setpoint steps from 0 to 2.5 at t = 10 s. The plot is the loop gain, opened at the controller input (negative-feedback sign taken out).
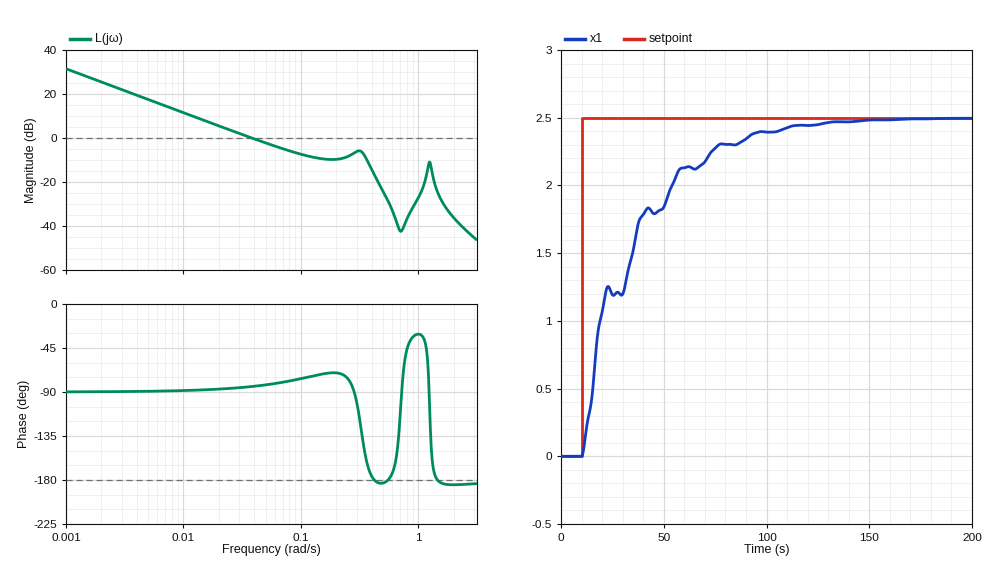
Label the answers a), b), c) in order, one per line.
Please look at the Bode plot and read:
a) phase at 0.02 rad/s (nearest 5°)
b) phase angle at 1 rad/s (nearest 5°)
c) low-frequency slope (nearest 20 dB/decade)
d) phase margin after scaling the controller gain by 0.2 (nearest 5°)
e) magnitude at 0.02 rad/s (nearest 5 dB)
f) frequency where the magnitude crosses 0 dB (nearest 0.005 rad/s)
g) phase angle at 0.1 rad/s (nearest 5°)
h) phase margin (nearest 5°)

a) -85°
b) -30°
c) -20 dB/decade
d) 90°
e) 5 dB
f) 0.040 rad/s
g) -75°
h) 95°
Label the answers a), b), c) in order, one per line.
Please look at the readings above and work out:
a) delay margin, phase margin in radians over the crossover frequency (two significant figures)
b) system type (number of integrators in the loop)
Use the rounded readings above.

a) 41 s
b) 1
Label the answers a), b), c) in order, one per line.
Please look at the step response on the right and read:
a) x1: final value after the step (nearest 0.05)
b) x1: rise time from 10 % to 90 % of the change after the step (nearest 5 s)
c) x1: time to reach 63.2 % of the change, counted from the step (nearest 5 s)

a) 2.50
b) 60 s
c) 25 s
